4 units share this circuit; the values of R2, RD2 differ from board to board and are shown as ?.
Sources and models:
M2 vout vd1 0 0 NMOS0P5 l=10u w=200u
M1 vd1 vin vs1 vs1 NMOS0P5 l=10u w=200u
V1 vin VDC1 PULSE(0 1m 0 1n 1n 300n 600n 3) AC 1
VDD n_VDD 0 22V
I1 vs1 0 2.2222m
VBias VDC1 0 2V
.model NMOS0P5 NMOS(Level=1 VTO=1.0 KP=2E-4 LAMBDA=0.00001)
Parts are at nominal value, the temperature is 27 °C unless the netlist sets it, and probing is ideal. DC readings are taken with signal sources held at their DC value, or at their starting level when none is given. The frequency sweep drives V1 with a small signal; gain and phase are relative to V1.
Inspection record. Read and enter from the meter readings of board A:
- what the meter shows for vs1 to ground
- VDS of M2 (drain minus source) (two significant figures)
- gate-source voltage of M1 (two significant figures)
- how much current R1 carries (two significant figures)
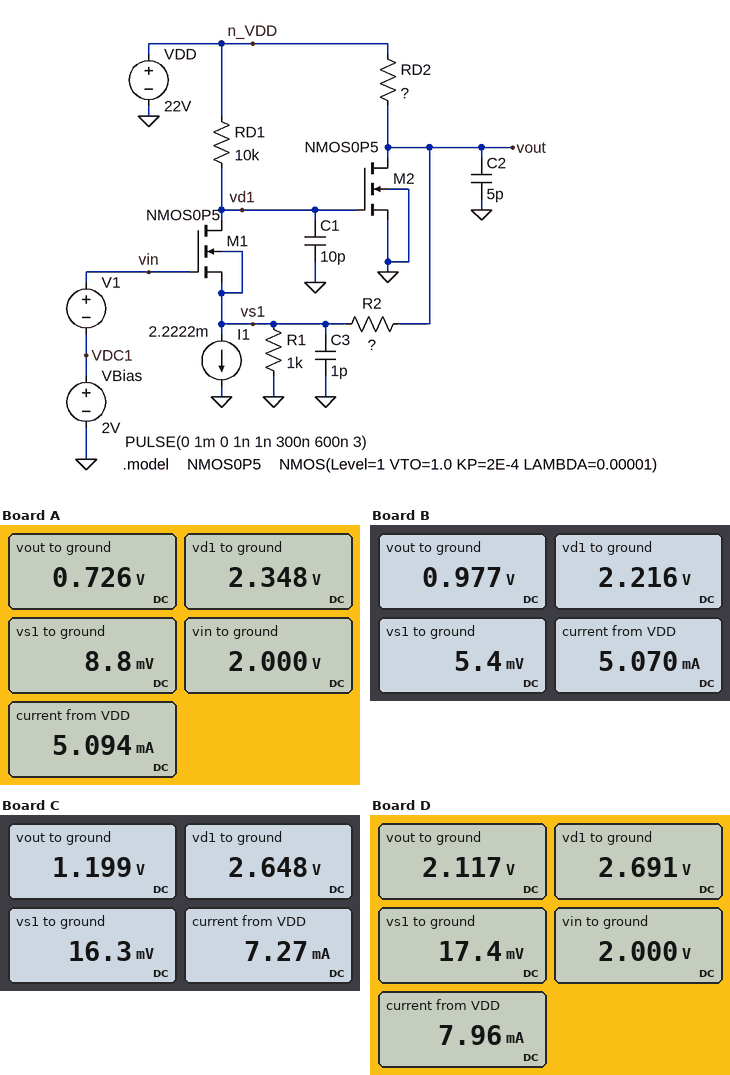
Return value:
8.8 mV
730 mV
2.0 V
8.8 µA
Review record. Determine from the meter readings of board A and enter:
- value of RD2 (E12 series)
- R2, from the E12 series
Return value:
6.8 kΩ
2.7 kΩ
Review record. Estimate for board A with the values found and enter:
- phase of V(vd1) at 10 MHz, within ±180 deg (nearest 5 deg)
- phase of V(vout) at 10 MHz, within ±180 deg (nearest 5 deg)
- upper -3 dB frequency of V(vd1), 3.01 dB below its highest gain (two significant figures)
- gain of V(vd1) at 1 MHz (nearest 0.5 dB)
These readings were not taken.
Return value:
125 deg
-60 deg
6.2 MHz
8.5 dB
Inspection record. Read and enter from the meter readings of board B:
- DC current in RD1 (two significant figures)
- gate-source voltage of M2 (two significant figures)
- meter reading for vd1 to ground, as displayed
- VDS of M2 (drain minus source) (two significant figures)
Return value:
2.0 mA
2.2 V
2.216 V
980 mV
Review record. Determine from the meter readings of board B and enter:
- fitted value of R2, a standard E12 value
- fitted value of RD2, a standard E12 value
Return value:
3.9 kΩ
6.8 kΩ
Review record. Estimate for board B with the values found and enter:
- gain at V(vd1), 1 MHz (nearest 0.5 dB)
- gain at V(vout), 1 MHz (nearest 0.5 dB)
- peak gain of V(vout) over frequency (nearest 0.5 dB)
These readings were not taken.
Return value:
3.0 dB
12.5 dB
12.5 dB
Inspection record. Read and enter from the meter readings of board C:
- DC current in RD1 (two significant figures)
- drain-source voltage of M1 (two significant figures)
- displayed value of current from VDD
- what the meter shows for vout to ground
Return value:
1.9 mA
2.6 V
7.27 mA
1.199 V
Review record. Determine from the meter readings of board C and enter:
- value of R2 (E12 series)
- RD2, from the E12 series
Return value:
3.9 kΩ
3.9 kΩ
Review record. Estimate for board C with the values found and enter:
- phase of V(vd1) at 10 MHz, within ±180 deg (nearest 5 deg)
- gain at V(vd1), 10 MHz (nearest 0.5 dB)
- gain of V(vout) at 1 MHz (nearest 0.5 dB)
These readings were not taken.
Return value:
135 deg
2.0 dB
12.0 dB
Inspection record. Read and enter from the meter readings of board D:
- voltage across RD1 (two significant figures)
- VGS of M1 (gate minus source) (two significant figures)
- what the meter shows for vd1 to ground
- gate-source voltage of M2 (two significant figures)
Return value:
19 V
2.0 V
2.691 V
2.7 V
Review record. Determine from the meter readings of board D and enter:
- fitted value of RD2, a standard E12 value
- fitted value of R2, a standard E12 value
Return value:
3.3 kΩ
6.8 kΩ
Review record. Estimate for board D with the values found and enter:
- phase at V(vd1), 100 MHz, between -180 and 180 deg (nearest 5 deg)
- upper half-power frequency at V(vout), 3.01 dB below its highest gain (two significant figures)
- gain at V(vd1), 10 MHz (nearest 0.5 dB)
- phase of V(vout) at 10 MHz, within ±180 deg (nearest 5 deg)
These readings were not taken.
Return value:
115 deg
24 MHz
-3.0 dB
-25 deg
